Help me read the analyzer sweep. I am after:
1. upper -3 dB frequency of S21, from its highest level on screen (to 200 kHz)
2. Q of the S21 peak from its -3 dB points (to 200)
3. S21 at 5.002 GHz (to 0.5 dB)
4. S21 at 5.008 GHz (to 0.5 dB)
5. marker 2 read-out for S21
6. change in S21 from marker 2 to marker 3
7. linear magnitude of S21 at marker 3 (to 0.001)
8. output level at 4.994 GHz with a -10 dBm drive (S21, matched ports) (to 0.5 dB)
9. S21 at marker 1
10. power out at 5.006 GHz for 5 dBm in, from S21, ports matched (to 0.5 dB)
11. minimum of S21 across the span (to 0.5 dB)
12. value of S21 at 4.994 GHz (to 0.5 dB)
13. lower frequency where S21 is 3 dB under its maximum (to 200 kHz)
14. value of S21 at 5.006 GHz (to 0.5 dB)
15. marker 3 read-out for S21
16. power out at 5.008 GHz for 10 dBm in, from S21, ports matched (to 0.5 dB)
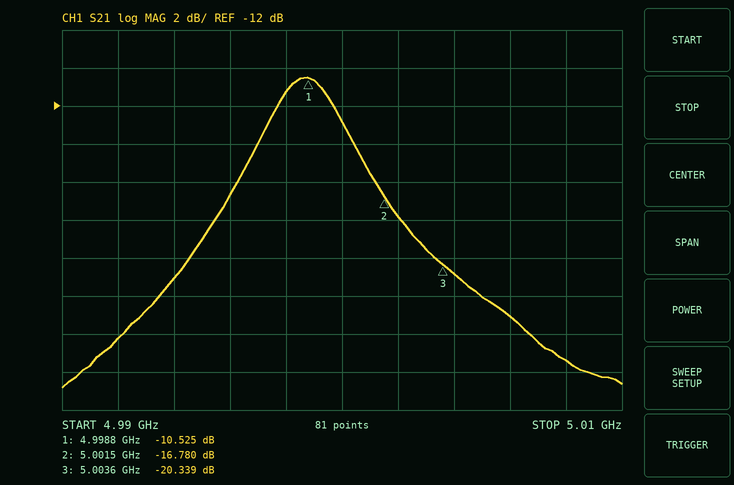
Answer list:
5.0002 GHz
1600
-18.0 dB
-25.5 dB
-16.780 dB
-3.559 dB
0.096
-31.0 dBm
-10.525 dB
-18.0 dBm
-27.0 dB
-21.0 dB
4.9972 GHz
-23.0 dB
-20.339 dB
-15.5 dBm
